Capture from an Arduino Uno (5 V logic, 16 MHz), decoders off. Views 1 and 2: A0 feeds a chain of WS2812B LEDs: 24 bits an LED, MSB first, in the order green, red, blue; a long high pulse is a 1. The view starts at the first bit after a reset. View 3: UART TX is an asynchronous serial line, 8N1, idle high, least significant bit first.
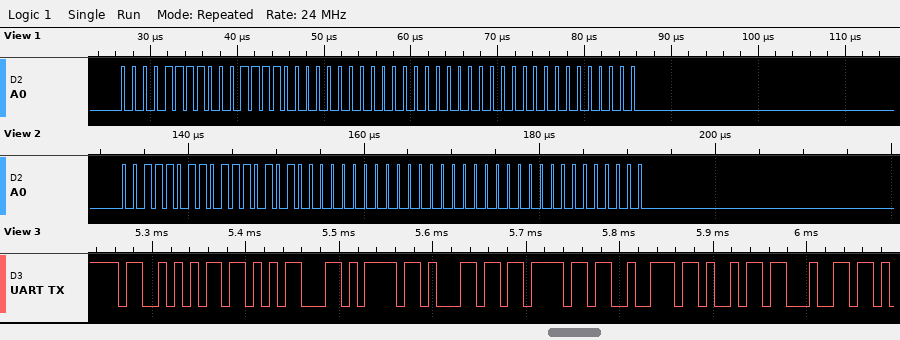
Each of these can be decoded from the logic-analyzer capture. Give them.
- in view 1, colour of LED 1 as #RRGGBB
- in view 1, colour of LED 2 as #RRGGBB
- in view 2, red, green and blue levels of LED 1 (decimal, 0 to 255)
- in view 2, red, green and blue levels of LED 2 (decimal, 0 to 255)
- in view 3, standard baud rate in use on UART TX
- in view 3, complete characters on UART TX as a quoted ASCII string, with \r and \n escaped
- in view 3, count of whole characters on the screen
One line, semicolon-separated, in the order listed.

#1E0F00; #000000; 117, 59, 0; 0, 0, 0; 115200 baud; "S[colorid"; 9
